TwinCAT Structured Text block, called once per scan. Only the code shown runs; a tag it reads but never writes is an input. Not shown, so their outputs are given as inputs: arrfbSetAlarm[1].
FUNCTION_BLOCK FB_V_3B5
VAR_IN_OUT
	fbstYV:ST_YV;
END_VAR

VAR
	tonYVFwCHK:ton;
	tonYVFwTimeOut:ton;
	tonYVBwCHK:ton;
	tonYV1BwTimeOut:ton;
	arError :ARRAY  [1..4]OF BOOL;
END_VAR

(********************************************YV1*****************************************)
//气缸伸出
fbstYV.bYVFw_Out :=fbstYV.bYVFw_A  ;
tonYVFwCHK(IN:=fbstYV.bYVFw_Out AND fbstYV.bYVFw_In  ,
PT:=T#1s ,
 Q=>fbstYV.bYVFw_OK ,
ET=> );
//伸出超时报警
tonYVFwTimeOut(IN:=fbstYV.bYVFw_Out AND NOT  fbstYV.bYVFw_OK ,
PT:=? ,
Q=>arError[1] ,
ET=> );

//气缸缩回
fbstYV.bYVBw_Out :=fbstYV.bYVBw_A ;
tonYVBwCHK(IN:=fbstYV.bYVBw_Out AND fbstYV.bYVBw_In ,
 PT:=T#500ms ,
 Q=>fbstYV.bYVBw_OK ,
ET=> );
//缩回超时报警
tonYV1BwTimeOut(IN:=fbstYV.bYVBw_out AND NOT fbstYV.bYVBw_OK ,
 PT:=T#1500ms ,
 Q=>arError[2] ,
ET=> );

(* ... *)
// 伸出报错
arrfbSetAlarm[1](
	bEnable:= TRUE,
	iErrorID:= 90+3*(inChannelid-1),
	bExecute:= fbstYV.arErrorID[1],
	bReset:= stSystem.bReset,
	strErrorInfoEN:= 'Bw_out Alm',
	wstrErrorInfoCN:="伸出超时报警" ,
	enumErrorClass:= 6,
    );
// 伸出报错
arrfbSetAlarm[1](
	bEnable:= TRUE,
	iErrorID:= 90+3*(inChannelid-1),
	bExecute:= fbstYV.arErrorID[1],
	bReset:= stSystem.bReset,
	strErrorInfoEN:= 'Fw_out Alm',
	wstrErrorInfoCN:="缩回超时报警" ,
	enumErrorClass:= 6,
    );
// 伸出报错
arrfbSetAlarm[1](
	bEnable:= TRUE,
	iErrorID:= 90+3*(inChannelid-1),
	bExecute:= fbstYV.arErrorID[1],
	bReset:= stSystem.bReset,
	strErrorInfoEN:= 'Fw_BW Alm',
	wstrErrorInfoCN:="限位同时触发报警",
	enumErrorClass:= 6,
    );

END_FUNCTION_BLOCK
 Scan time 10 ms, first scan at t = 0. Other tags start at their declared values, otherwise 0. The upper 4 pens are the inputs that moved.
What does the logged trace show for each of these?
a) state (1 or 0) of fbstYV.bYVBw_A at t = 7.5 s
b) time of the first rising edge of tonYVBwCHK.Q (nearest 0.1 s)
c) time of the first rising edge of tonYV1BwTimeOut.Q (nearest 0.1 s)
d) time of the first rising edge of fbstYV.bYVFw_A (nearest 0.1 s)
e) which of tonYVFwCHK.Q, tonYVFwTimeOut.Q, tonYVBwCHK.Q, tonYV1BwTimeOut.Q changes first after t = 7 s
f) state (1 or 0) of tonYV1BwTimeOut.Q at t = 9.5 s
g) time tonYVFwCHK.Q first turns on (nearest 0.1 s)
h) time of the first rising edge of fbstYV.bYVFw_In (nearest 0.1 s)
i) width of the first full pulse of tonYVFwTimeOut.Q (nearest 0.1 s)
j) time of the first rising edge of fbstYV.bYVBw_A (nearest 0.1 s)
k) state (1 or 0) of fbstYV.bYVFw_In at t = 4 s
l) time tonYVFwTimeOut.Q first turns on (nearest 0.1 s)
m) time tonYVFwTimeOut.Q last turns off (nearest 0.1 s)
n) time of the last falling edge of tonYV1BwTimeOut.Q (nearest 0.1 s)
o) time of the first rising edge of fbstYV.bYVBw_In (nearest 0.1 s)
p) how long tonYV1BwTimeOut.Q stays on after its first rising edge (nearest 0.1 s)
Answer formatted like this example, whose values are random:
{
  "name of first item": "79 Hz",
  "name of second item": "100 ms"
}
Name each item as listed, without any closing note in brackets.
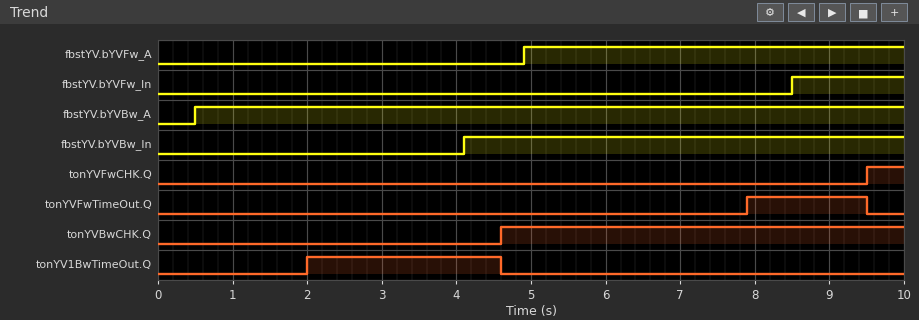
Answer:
{
  "state (1 or 0) of fbstYV.bYVBw_A at t = 7.5 s": "1",
  "time of the first rising edge of tonYVBwCHK.Q": "4.6 s",
  "time of the first rising edge of tonYV1BwTimeOut.Q": "2.0 s",
  "time of the first rising edge of fbstYV.bYVFw_A": "4.9 s",
  "which of tonYVFwCHK.Q, tonYVFwTimeOut.Q, tonYVBwCHK.Q, tonYV1BwTimeOut.Q changes first after t = 7 s": "tonYVFwTimeOut.Q",
  "state (1 or 0) of tonYV1BwTimeOut.Q at t = 9.5 s": "0",
  "time tonYVFwCHK.Q first turns on": "9.5 s",
  "time of the first rising edge of fbstYV.bYVFw_In": "8.5 s",
  "width of the first full pulse of tonYVFwTimeOut.Q": "1.6 s",
  "time of the first rising edge of fbstYV.bYVBw_A": "0.5 s",
  "state (1 or 0) of fbstYV.bYVFw_In at t = 4 s": "0",
  "time tonYVFwTimeOut.Q first turns on": "7.9 s",
  "time tonYVFwTimeOut.Q last turns off": "9.5 s",
  "time of the last falling edge of tonYV1BwTimeOut.Q": "4.6 s",
  "time of the first rising edge of fbstYV.bYVBw_In": "4.1 s",
  "how long tonYV1BwTimeOut.Q stays on after its first rising edge": "2.6 s"
}
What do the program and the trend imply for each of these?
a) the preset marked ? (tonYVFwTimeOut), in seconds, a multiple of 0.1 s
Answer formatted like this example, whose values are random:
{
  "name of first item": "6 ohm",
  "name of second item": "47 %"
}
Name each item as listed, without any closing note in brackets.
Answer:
{
  "the preset marked ? (tonYVFwTimeOut), in seconds, a multiple of 0.1 s": "3.0 s"
}
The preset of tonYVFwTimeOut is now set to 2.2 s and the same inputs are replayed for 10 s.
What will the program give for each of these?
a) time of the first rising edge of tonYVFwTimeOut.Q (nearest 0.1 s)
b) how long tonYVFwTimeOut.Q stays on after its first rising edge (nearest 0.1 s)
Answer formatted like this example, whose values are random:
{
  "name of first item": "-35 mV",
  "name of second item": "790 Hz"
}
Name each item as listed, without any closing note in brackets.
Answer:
{
  "time of the first rising edge of tonYVFwTimeOut.Q": "7.1 s",
  "how long tonYVFwTimeOut.Q stays on after its first rising edge": "2.4 s"
}
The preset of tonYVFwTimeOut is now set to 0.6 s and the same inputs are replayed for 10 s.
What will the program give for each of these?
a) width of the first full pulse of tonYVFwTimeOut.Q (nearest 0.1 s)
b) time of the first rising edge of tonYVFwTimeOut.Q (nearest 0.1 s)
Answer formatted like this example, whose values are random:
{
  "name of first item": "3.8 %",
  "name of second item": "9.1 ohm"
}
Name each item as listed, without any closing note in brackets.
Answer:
{
  "width of the first full pulse of tonYVFwTimeOut.Q": "4.0 s",
  "time of the first rising edge of tonYVFwTimeOut.Q": "5.5 s"
}
